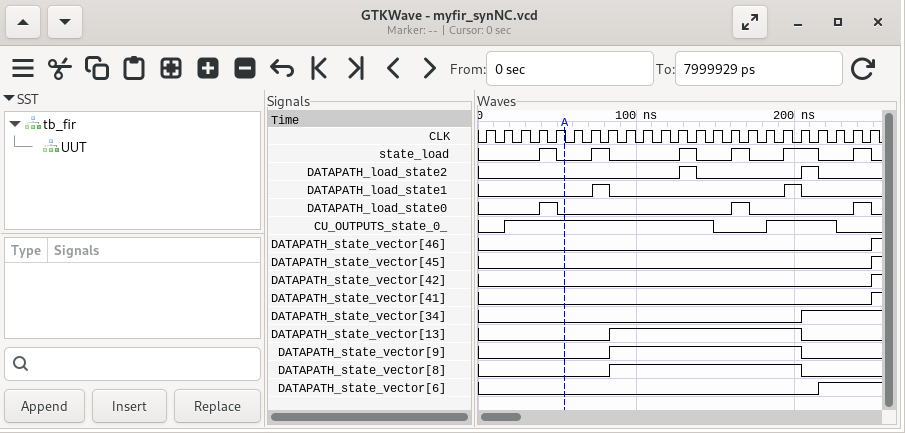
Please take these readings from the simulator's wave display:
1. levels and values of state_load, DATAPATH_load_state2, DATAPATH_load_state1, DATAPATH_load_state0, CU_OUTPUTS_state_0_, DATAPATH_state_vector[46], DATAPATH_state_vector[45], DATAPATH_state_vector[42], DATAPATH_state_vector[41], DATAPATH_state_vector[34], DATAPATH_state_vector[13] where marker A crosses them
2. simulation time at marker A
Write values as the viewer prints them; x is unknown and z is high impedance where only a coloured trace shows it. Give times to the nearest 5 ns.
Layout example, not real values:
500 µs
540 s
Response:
state_load=0, DATAPATH_load_state2=0, DATAPATH_load_state1=0, DATAPATH_load_state0=0, CU_OUTPUTS_state_0_=1, DATAPATH_state_vector[46]=0, DATAPATH_state_vector[45]=0, DATAPATH_state_vector[42]=0, DATAPATH_state_vector[41]=0, DATAPATH_state_vector[34]=0, DATAPATH_state_vector[13]=0
55 ns
